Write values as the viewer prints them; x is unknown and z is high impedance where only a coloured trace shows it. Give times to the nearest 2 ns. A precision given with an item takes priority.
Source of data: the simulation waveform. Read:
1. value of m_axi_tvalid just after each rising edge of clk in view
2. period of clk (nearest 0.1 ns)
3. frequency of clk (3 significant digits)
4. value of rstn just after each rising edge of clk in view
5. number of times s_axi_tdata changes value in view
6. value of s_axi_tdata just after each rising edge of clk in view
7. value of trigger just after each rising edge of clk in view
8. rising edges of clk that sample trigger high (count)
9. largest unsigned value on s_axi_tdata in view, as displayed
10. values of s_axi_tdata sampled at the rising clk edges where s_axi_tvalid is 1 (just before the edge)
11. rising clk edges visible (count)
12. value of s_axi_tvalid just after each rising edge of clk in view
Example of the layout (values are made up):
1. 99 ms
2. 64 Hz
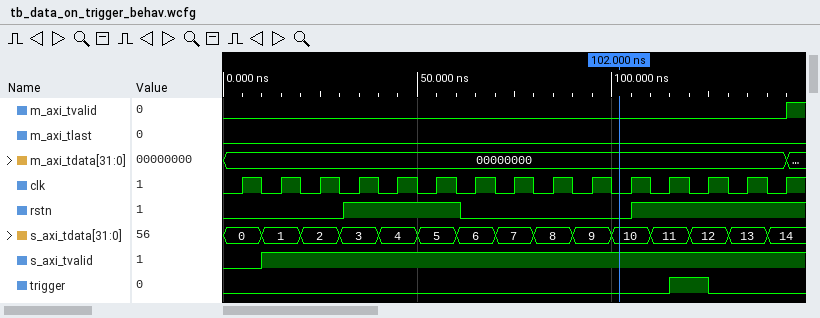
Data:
1. 0 0 0 0 0 0 0 0 0 0 0 0 0 0 1
2. 10 ns
3. 100 MHz
4. 0 0 0 1 1 1 0 0 0 0 1 1 1 1 1
5. 14
6. 0, 1, 2, 3, 4, 5, 6, 7, 8, 9, 10, 11, 12, 13, 14
7. 0 0 0 0 0 0 0 0 0 0 0 1 0 0 0
8. 1
9. 14
10. 1, 2, 3, 4, 5, 6, 7, 8, 9, 10, 11, 12, 13, 14
11. 15
12. 0 1 1 1 1 1 1 1 1 1 1 1 1 1 1
